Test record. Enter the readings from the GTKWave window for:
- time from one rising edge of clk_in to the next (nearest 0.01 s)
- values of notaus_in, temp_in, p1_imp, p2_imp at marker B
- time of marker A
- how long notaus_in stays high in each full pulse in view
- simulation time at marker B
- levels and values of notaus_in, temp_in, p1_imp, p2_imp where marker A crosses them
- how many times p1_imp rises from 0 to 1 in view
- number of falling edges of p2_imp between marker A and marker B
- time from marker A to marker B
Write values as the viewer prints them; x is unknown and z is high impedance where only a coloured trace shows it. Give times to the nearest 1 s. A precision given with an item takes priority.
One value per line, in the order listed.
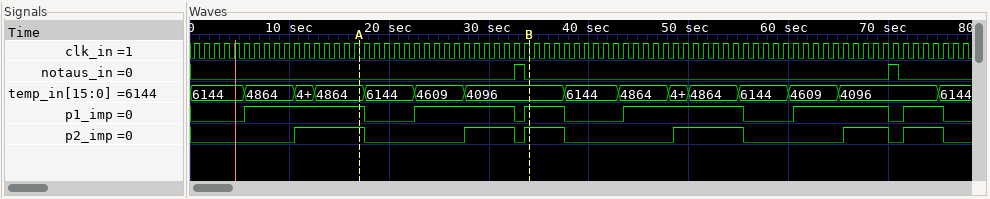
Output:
1 s
notaus_in=0, temp_in=4096, p1_imp=1, p2_imp=1
17 s
1 s, 1 s
34 s
notaus_in=0, temp_in=4864, p1_imp=1, p2_imp=1
6
2
17 s
